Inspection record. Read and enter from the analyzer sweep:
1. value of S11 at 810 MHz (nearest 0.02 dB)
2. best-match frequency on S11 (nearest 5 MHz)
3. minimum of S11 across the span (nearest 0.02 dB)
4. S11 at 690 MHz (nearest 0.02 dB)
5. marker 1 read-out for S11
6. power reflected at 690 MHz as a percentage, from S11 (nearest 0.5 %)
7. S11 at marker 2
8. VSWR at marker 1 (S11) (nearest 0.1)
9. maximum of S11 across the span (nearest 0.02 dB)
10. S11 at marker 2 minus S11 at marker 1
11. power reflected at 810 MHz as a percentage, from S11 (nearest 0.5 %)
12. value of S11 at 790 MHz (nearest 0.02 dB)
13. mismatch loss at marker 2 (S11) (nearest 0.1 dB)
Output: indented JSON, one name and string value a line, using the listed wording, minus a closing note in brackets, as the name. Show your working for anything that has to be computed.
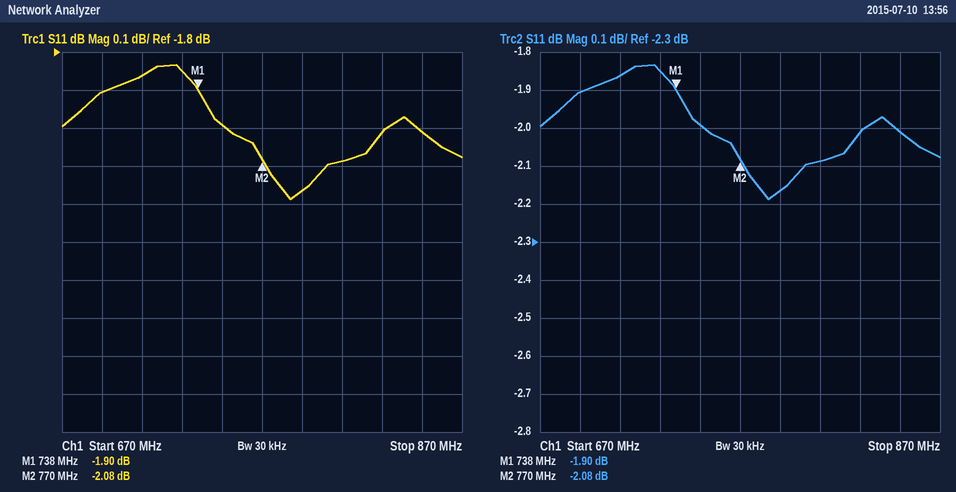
{
  "value of S11 at 810 MHz": "-2.08 dB",
  "best-match frequency on S11": "785 MHz",
  "minimum of S11 across the span": "-2.18 dB",
  "S11 at 690 MHz": "-1.90 dB",
  "marker 1 read-out for S11": "-1.90 dB",
  "power reflected at 690 MHz as a percentage, from S11": "10^(-1.9/10) ≈ 64.6 %, so 64.5 % to the nearest 0.5 %",
  "S11 at marker 2": "-2.08 dB",
  "VSWR at marker 1 (S11)": "(1 + 0.8035)/(1 − 0.8035) ≈ 9.2",
  "maximum of S11 across the span": "-1.84 dB",
  "S11 at marker 2 minus S11 at marker 1": "-2.08 − (-1.9) = -0.18 dB",
  "power reflected at 810 MHz as a percentage, from S11": "10^(-2.08/10) ≈ 61.9 %, so 62.0 % to the nearest 0.5 %",
  "value of S11 at 790 MHz": "-2.16 dB",
  "mismatch loss at marker 2 (S11)": "−10 log10(1 − 10^(-2.08/10)) ≈ 4.2 dB"
}
